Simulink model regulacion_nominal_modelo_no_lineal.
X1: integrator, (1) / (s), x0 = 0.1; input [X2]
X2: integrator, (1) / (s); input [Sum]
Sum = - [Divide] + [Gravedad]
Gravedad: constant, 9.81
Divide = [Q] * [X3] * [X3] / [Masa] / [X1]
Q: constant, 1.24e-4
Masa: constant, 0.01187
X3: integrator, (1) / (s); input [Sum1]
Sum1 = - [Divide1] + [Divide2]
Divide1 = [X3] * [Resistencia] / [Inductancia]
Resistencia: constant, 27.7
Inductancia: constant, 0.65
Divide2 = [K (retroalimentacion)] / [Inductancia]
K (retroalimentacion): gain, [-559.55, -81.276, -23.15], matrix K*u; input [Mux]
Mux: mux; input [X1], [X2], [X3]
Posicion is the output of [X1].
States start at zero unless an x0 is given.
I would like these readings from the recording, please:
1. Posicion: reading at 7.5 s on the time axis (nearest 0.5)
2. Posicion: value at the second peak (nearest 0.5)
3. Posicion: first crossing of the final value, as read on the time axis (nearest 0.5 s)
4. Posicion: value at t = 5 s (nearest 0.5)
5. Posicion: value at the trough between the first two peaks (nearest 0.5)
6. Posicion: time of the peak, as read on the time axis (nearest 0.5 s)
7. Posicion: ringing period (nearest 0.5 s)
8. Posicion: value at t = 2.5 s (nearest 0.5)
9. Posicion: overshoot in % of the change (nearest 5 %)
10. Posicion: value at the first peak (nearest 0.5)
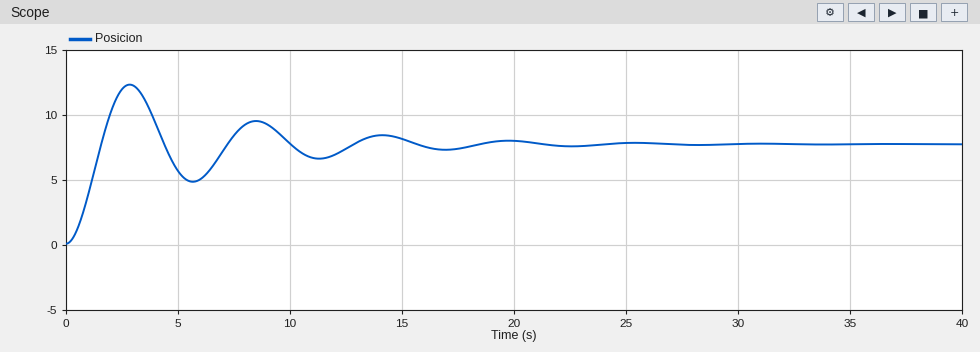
8.5
9.5
1.5 s
5.5
5.0
3.0 s
5.5 s
12.0
60 %
12.5
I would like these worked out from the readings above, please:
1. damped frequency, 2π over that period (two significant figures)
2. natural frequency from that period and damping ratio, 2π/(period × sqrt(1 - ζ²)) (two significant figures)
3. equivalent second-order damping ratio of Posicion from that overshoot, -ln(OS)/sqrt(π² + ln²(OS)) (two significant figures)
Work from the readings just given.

1.1 rad/s
1.2 rad/s
0.16
